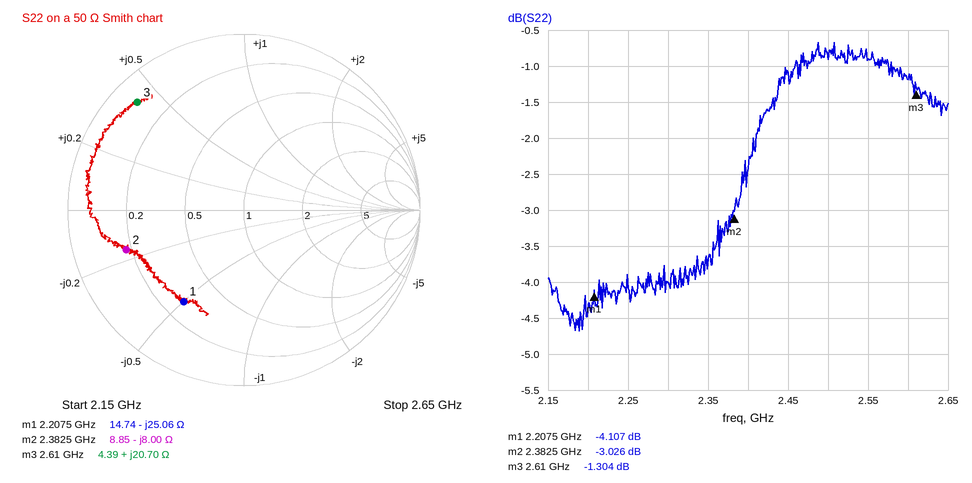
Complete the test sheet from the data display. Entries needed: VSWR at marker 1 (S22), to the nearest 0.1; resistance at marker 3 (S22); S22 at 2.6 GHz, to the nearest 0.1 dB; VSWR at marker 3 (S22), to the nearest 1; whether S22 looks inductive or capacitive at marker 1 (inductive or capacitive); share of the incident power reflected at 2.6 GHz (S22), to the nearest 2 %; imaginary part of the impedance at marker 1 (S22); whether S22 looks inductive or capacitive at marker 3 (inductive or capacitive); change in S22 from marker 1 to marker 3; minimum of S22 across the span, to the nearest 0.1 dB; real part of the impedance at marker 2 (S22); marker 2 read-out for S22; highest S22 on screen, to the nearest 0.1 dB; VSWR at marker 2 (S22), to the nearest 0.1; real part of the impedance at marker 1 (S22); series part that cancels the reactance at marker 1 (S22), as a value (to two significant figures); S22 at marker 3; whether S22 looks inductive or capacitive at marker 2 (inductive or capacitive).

4.3
4.39 Ω
-1.2 dB
13
capacitive
76 %
-25.06 Ω
inductive
2.803 dB
-4.7 dB
8.85 Ω
-3.026 dB
-0.7 dB
5.8
14.74 Ω
1.8 nH
-1.304 dB
capacitive
